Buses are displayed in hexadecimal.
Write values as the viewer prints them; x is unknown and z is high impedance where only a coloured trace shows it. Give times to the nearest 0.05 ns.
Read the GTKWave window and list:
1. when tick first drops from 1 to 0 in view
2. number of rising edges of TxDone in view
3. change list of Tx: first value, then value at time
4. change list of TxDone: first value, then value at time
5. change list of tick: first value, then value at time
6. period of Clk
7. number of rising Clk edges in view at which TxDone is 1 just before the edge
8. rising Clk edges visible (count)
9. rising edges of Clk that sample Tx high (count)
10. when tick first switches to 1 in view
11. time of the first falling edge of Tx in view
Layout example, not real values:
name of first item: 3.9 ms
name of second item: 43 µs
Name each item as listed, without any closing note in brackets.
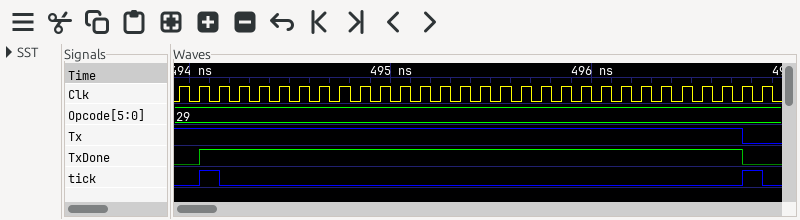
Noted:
when tick first drops from 1 to 0 in view: 494.15 ns
number of rising edges of TxDone in view: 1
change list of Tx: first value, then value at time: 1, 0 at 496.75 ns
change list of TxDone: first value, then value at time: 0, 1 at 494.05 ns, 0 at 496.75 ns
change list of tick: first value, then value at time: 0, 1 at 494.05 ns, 0 at 494.15 ns, 1 at 496.75 ns, 0 at 496.85 ns
period of Clk: 0.1 ns
number of rising Clk edges in view at which TxDone is 1 just before the edge: 27
rising Clk edges visible: 30
rising edges of Clk that sample Tx high: 29
when tick first switches to 1 in view: 494.05 ns
time of the first falling edge of Tx in view: 496.75 ns
